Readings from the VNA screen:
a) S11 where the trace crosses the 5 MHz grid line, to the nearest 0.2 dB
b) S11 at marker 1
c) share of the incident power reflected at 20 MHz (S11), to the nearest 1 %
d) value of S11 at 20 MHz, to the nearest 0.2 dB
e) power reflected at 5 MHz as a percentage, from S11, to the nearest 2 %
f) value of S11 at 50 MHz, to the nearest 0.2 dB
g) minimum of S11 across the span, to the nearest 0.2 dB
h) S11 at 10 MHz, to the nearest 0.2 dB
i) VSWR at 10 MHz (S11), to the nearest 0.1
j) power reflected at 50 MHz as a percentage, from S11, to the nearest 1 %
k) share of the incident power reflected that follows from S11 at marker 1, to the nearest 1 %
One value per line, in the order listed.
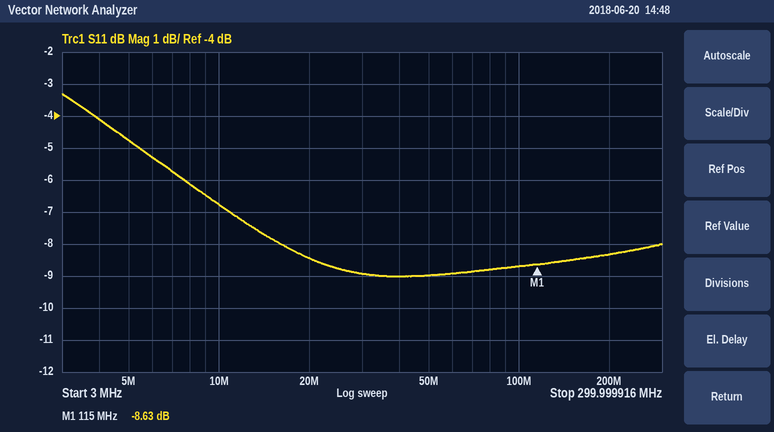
-4.8 dB
-8.63 dB
14 %
-8.4 dB
34 %
-9.0 dB
-9.0 dB
-6.8 dB
2.7
13 %
14 %
